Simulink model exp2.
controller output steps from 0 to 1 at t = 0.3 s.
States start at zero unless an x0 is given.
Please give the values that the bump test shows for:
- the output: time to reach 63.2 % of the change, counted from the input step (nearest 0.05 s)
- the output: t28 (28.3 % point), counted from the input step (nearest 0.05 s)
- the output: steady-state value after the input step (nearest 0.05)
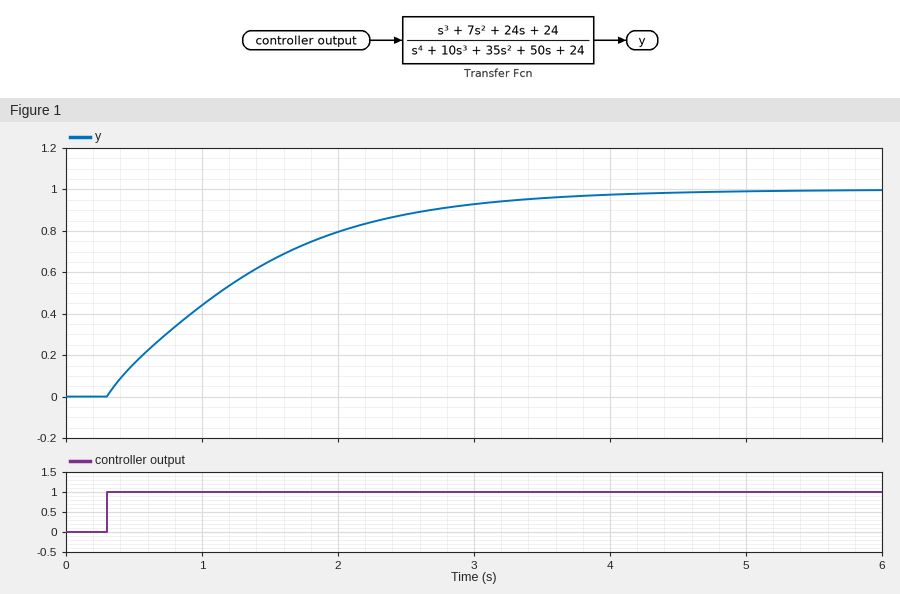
1.15 s
0.40 s
1.00
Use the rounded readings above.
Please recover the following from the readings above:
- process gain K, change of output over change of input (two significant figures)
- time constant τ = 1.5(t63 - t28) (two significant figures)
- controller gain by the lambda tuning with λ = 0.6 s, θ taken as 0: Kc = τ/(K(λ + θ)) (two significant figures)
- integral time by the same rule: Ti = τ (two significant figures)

1.0
1.1 s
1.8
1.1 s
